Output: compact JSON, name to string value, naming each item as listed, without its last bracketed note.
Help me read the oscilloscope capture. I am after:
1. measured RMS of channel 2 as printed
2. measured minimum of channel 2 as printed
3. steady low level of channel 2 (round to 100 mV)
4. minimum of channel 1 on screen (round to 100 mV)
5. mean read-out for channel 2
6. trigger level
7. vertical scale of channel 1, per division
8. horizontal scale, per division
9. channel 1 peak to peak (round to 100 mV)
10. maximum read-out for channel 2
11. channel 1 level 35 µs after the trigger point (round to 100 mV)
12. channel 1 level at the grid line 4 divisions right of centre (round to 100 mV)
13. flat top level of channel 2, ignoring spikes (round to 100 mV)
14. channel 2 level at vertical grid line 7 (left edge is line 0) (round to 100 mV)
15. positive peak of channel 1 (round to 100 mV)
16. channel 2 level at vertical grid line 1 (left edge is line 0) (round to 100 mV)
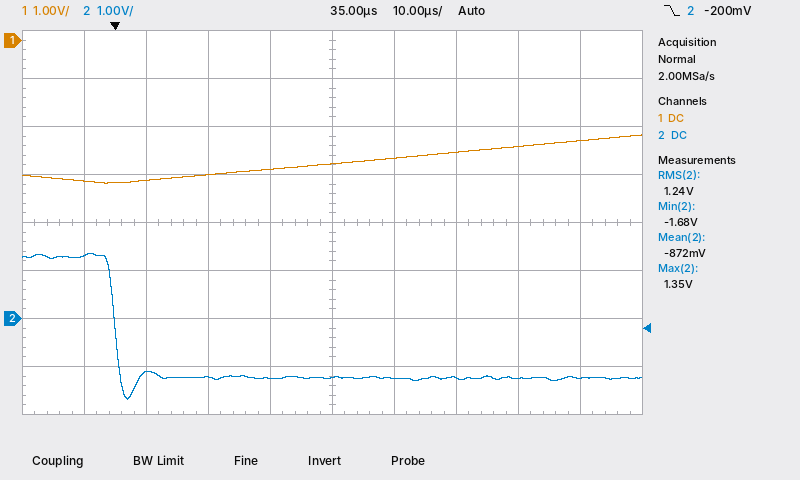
{"measured RMS of channel 2 as printed": "1.24 V", "measured minimum of channel 2 as printed": "-1.68 V", "steady low level of channel 2": "-1.2 V", "minimum of channel 1 on screen": "-3.0 V", "mean read-out for channel 2": "-872 mV", "trigger level": "-200 mV", "vertical scale of channel 1, per division": "1 V", "horizontal scale, per division": "10 µs", "channel 1 peak to peak": "1.0 V", "maximum read-out for channel 2": "1.35 V", "channel 1 level 35 µs after the trigger point": "-2.6 V", "channel 1 level at the grid line 4 divisions right of centre": "-2.1 V", "flat top level of channel 2, ignoring spikes": "1.3 V", "channel 2 level at vertical grid line 7 (left edge is line 0)": "-1.2 V", "positive peak of channel 1": "-2.0 V", "channel 2 level at vertical grid line 1 (left edge is line 0)": "1.3 V"}
